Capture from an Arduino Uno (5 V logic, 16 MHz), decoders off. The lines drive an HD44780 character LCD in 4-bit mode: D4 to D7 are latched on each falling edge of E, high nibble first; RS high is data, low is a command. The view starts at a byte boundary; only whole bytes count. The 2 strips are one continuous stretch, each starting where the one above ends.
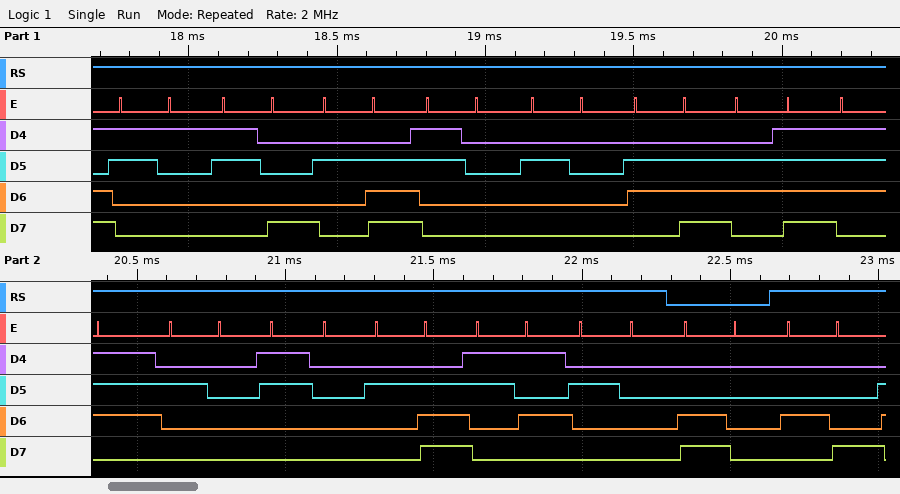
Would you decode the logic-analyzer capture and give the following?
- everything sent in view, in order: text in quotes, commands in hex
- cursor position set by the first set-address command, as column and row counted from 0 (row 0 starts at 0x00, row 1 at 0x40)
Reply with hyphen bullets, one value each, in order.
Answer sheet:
- "18.0 now 0.5 " 0xC0 "H"
- column 0, row 1
